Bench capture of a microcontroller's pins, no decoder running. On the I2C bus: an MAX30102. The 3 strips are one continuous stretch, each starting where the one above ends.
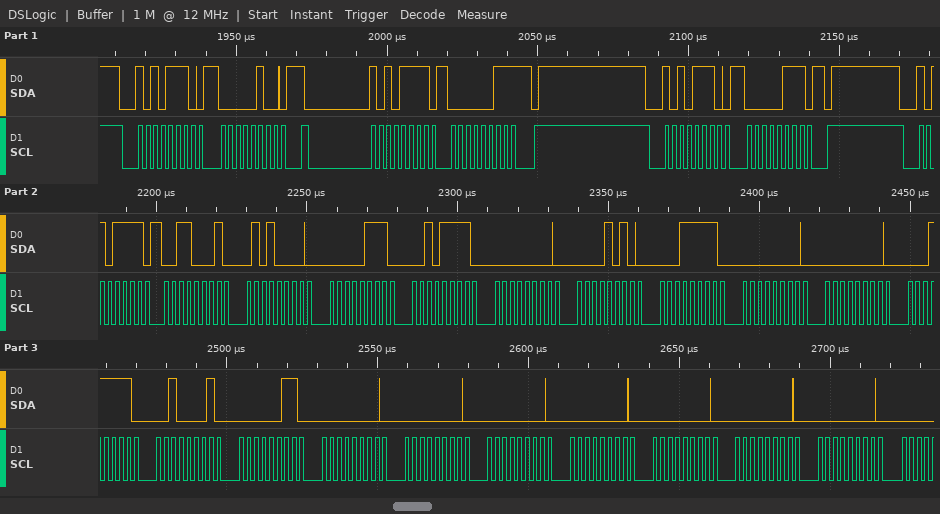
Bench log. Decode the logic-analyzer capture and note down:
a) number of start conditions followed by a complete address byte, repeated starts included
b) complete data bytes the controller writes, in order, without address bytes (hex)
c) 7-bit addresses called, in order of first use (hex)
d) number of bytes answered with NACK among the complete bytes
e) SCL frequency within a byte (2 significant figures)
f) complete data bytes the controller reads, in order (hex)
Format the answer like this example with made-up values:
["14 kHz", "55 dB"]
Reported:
["4", "04 07", "0x57", "1", "400 kHz", "03 31 50 07 2F 00 0A 1F 00 00 1F 21 03 00 00 00 00 00 00 00"]
